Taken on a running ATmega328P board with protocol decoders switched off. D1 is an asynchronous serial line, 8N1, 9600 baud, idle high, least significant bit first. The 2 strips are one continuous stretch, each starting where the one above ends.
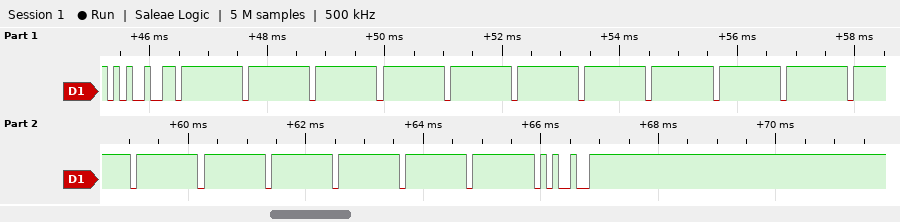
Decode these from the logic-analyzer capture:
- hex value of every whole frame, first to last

0x25 0xFF 0xFF 0xFF 0xFF 0xFF 0xFF 0xFF 0xFF 0xFF 0xFF 0xFF 0xFF 0xFF 0xFF 0xFF 0xFF 0xFF 0x25
